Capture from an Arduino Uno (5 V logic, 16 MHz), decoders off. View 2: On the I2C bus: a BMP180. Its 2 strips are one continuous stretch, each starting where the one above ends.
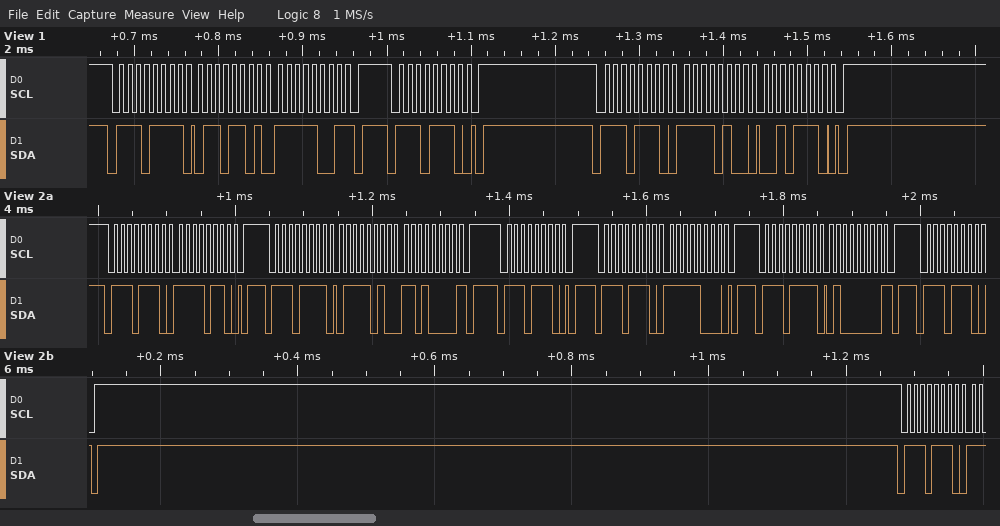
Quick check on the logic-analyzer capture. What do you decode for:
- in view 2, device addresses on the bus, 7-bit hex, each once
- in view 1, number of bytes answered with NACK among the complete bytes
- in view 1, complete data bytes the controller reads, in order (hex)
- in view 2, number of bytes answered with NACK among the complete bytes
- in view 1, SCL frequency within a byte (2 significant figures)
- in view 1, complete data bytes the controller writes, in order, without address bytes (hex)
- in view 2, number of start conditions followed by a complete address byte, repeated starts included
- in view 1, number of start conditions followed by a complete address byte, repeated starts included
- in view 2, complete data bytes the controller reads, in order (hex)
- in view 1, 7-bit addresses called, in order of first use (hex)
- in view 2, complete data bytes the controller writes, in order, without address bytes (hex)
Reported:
0x77
1
6D F9
2
100 kHz
F4 2E
7
3
7A D0 40
0x77
F6 F8
